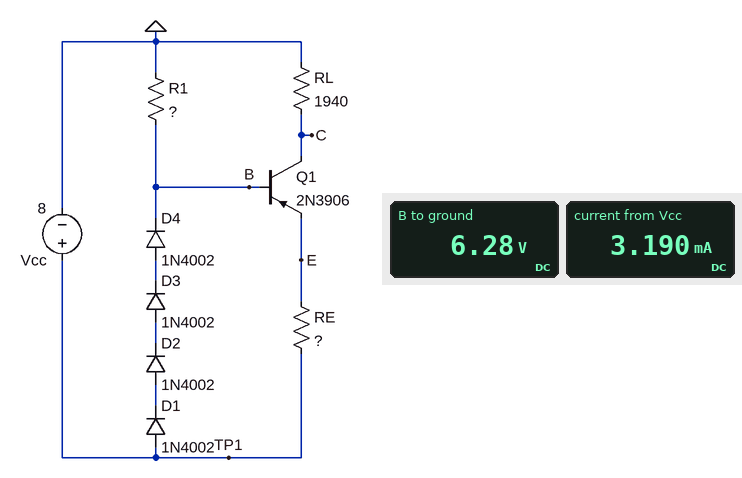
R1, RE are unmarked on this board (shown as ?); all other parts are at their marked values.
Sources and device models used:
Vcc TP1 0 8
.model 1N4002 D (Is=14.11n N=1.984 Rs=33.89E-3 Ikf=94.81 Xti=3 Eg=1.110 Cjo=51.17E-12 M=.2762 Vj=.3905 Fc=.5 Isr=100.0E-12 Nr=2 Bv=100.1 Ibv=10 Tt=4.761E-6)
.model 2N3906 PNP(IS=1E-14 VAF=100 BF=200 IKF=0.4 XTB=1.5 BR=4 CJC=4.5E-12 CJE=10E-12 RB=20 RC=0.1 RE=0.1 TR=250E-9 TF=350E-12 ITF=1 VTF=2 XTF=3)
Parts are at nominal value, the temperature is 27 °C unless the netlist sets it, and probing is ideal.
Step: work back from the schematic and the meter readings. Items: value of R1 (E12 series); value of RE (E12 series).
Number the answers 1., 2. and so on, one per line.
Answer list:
1. 82 kΩ
2. 330 Ω
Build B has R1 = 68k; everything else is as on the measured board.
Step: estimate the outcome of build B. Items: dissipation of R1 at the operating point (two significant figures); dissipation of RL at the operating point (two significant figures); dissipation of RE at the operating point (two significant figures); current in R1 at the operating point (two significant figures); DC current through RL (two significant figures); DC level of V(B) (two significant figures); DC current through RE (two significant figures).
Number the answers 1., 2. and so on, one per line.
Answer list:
1. 570 µW
2. 20 mW
3. 3.5 mW
4. 92 µA
5. 3.2 mA
6. 6.2 V
7. 3.3 mA
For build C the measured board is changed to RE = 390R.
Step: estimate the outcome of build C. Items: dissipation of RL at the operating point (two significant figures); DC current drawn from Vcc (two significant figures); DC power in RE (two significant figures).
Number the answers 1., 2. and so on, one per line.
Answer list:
1. 14 mW
2. 2.7 mA
3. 2.8 mW
